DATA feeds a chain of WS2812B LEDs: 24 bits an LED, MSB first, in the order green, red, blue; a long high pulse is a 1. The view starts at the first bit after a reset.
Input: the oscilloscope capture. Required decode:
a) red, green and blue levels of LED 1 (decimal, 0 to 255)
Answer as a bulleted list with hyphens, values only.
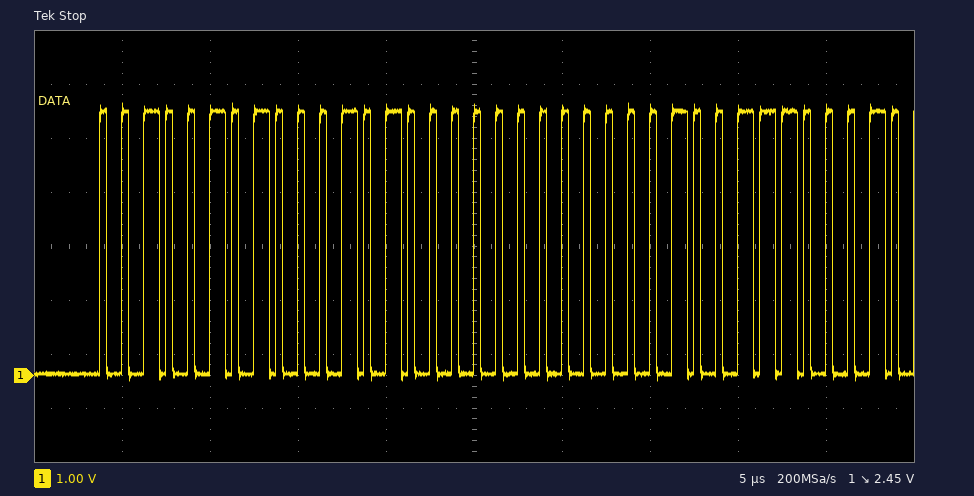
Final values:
- 20, 37, 0
